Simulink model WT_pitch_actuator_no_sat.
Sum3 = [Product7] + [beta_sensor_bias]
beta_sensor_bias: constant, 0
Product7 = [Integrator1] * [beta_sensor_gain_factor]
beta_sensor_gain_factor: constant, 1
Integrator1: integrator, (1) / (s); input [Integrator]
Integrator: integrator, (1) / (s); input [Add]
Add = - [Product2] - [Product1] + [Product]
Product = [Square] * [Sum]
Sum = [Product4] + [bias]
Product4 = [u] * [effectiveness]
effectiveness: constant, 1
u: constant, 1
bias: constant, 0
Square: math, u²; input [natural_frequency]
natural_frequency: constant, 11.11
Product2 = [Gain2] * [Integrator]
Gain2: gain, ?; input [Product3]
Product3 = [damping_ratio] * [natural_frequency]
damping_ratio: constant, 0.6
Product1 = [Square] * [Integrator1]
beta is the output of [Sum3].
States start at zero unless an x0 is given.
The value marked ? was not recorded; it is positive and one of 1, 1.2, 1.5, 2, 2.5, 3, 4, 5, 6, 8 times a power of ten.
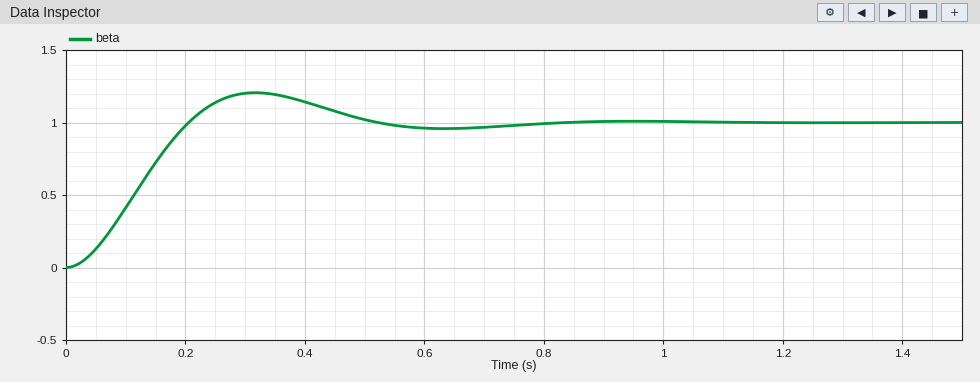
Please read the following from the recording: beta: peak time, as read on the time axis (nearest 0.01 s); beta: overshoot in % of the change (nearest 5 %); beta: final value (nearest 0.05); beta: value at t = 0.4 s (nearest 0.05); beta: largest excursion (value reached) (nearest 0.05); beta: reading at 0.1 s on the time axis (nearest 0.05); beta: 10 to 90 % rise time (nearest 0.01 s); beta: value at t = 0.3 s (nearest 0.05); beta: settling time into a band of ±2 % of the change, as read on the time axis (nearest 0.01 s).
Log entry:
0.32 s
20 %
1.00
1.15
1.20
0.40
0.14 s
1.20
0.75 s
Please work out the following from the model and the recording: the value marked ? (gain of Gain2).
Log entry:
1.5
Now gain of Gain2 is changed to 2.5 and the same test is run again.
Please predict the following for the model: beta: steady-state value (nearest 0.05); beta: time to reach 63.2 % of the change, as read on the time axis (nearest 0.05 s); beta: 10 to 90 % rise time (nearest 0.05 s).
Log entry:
1.00
0.15 s
0.20 s
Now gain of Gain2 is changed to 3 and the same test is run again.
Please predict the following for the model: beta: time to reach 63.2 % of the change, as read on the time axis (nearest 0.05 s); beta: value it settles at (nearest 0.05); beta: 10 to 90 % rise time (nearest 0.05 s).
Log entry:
0.20 s
1.00
0.25 s
